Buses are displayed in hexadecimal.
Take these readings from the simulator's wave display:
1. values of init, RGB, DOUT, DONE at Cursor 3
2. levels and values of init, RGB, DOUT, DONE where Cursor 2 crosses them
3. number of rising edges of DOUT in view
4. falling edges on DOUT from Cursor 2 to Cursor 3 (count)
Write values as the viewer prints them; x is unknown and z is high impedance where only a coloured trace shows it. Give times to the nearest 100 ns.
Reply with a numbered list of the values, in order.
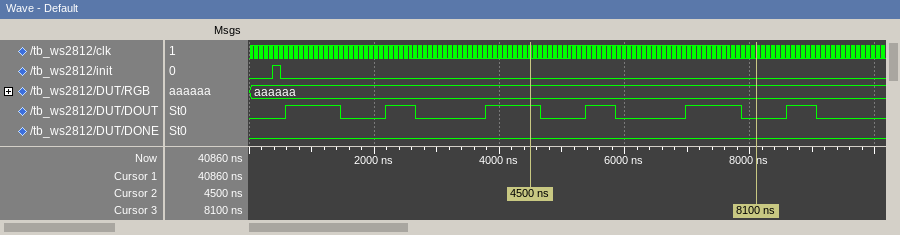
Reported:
1. init=0, RGB=aaaaaa, DOUT=0, DONE=0
2. init=0, RGB=aaaaaa, DOUT=1, DONE=0
3. 6
4. 3
